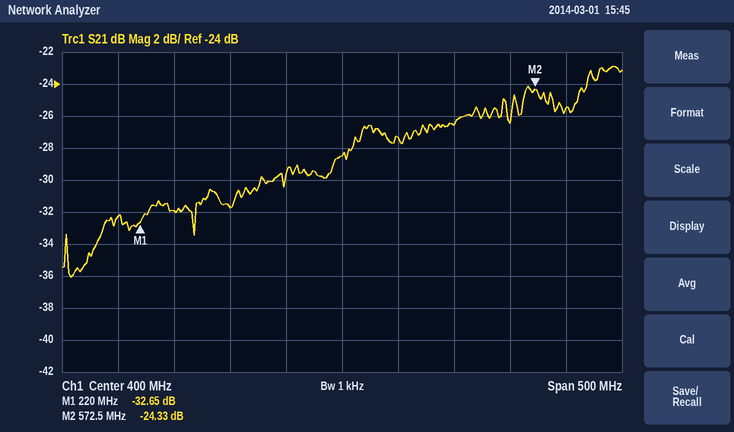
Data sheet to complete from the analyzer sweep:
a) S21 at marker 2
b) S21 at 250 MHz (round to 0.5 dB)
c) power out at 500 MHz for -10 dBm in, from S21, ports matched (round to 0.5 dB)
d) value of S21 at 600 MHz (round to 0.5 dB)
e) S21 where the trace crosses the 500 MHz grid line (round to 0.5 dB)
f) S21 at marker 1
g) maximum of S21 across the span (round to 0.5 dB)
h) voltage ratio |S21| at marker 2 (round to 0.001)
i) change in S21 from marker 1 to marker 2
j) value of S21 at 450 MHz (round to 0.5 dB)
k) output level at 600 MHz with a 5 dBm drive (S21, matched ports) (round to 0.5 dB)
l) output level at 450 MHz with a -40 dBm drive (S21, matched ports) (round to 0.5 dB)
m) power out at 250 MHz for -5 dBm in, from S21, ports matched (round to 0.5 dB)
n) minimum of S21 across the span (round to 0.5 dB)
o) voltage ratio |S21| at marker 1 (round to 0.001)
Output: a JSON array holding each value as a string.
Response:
["-24.33 dB", "-32.0 dB", "-36.5 dBm", "-25.5 dB", "-26.5 dB", "-32.65 dB", "-23.0 dB", "0.061", "8.32 dB", "-27.5 dB", "-20.5 dBm", "-67.5 dBm", "-37.0 dBm", "-36.0 dB", "0.023"]
